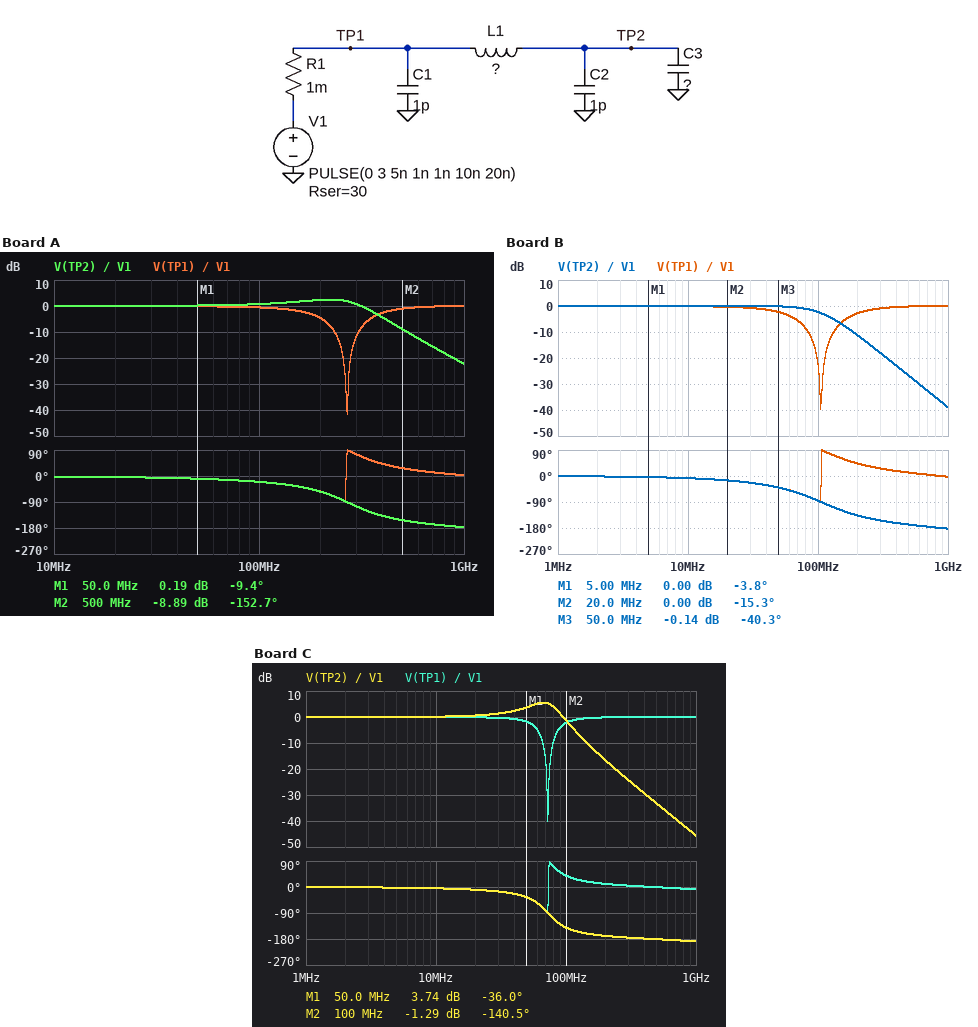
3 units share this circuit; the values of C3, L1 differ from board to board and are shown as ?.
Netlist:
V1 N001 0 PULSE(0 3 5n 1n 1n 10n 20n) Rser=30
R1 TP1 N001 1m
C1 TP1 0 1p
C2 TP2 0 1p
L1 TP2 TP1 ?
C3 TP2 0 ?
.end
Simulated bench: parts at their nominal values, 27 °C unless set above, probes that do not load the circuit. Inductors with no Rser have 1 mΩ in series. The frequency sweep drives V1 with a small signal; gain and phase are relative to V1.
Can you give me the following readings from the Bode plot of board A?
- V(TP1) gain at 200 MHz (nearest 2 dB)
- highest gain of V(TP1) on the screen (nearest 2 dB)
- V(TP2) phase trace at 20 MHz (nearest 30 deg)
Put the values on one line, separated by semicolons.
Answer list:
-4 dB; 0 dB; 0 deg
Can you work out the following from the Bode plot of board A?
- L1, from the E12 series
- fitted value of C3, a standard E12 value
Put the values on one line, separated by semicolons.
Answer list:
22 nH; 15 pF
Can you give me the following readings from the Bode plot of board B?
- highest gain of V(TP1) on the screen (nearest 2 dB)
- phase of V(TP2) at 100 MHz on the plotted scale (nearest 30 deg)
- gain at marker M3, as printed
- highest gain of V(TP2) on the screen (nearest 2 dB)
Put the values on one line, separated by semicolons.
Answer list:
0 dB; -90 deg; -0.14 dB; 0 dB
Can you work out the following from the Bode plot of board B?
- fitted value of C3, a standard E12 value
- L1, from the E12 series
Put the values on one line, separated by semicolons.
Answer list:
68 pF; 33 nH
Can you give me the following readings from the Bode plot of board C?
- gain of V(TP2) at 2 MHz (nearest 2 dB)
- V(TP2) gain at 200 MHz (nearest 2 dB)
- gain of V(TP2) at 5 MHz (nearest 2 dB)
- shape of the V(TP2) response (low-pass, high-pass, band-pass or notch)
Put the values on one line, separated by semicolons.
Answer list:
0 dB; -16 dB; 0 dB; low-pass
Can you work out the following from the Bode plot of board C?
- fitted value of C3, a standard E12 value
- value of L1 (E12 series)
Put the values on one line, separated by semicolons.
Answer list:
39 pF; 120 nH
